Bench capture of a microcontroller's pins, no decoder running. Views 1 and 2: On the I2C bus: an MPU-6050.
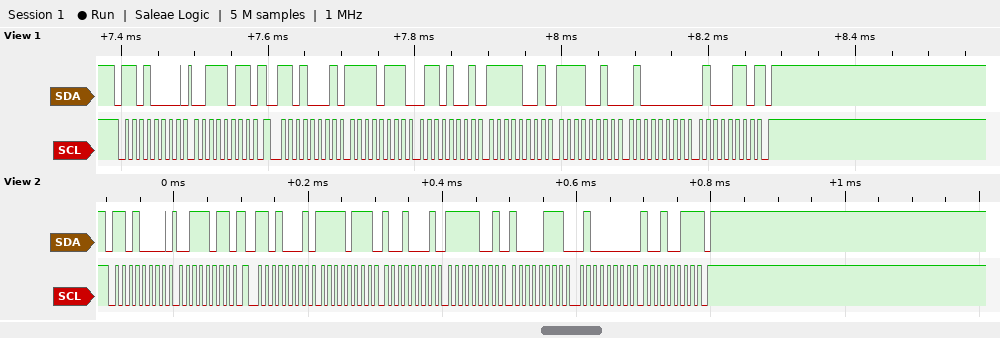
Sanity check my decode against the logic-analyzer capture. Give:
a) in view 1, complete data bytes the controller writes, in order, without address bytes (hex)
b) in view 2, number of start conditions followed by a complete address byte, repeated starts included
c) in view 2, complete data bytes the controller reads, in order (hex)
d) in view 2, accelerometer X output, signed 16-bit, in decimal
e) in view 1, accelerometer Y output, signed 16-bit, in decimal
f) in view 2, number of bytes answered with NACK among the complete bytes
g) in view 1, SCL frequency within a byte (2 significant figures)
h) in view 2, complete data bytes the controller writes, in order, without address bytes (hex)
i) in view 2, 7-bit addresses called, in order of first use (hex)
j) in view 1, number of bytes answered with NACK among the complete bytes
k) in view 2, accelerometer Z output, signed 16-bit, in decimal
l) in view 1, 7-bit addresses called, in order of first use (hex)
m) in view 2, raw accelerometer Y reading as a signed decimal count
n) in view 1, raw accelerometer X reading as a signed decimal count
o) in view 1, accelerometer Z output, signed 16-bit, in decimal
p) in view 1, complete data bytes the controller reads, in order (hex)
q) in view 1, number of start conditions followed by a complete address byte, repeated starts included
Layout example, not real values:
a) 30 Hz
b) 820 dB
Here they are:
a) 3B
b) 2
c) F7 91 F9 87 40 93
d) -2159
e) -1550
f) 1
g) 100 kHz
h) 3B
i) 0x68
j) 1
k) 16531
l) 0x68
m) -1657
n) -2199
o) 16454
p) F7 69 F9 F2 40 46
q) 2
